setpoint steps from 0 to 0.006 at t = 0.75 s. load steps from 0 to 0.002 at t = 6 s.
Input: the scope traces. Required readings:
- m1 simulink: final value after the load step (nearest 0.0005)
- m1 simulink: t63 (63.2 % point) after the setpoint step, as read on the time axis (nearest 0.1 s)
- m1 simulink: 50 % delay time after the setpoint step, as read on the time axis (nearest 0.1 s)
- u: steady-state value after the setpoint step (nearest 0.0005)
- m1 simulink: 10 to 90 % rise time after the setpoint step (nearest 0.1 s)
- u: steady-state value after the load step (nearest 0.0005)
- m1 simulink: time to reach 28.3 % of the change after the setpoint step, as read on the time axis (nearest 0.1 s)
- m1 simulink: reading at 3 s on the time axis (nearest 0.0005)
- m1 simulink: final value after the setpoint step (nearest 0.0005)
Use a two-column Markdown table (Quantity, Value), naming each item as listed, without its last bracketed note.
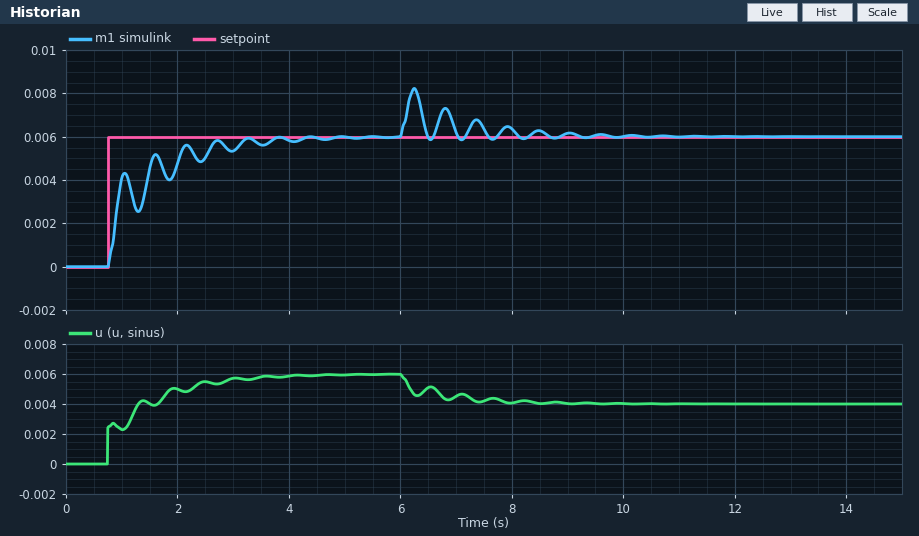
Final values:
| Quantity | Value |
|---|---|
| m1 simulink: final value after the load step | 0.0060 |
| m1 simulink: t63 (63.2 % point) after the setpoint step, as read on the time axis | 1.0 s |
| m1 simulink: 50 % delay time after the setpoint step, as read on the time axis | 0.9 s |
| u: steady-state value after the setpoint step | 0.0060 |
| m1 simulink: 10 to 90 % rise time after the setpoint step | 1.3 s |
| u: steady-state value after the load step | 0.0040 |
| m1 simulink: time to reach 28.3 % of the change after the setpoint step, as read on the time axis | 0.9 s |
| m1 simulink: reading at 3 s on the time axis | 0.0055 |
| m1 simulink: final value after the setpoint step | 0.0060 |
